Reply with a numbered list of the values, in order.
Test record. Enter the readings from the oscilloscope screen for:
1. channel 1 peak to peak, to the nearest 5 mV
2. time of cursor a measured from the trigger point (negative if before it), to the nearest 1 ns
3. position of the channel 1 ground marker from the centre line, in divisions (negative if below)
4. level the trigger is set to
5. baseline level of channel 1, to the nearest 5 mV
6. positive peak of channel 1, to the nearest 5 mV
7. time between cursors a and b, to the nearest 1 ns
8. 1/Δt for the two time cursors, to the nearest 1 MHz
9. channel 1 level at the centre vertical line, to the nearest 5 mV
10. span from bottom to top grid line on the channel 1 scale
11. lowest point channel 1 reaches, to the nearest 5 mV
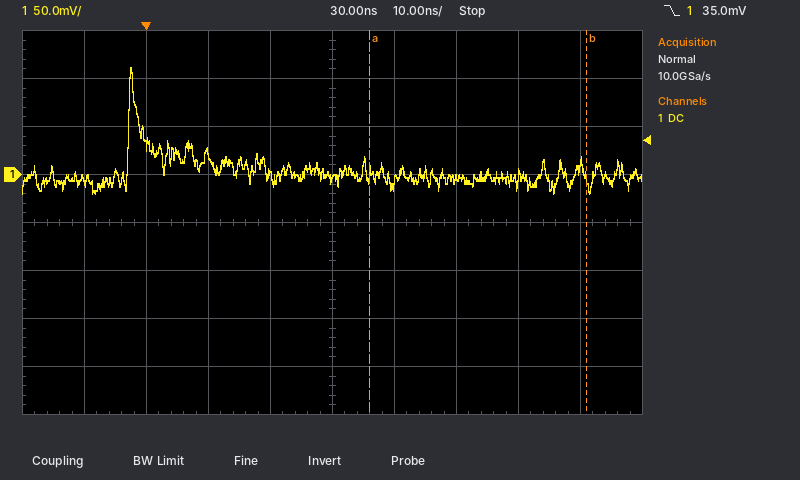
1. 130 mV
2. +36 ns
3. +1.0 div
4. 35.0 mV
5. 0 mV
6. 110 mV
7. 35 ns
8. 29 MHz
9. -5 mV
10. 400 mV
11. -20 mV
